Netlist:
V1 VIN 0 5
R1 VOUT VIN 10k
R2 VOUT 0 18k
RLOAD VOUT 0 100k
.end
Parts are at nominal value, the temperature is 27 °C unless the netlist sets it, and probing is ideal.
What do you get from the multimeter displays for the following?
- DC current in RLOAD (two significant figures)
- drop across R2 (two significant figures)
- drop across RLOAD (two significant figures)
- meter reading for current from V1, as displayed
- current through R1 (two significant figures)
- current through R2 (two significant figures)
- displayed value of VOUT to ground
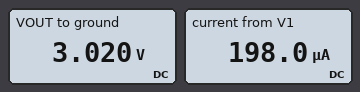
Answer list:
30 µA
3.0 V
3.0 V
198.0 µA
200 µA
170 µA
3.020 V
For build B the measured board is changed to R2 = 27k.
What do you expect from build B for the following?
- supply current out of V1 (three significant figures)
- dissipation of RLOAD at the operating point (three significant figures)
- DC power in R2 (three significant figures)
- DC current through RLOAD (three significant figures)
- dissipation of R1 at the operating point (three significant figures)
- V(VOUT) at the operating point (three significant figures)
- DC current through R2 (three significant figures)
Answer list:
160 µA
116 µW
428 µW
34.0 µA
256 µW
3.40 V
126 µA
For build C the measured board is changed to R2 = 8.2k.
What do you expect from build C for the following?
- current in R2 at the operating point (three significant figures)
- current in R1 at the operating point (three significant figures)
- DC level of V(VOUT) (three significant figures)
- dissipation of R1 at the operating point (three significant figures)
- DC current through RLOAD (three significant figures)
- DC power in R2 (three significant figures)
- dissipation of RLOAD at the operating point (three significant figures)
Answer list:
263 µA
284 µA
2.16 V
809 µW
21.6 µA
567 µW
46.5 µW
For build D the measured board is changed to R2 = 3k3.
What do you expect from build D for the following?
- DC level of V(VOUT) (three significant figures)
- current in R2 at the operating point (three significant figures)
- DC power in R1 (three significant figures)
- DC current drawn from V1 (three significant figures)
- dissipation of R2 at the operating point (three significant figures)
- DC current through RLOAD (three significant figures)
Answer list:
1.21 V
367 µA
1.44 mW
379 µA
444 µW
12.1 µA
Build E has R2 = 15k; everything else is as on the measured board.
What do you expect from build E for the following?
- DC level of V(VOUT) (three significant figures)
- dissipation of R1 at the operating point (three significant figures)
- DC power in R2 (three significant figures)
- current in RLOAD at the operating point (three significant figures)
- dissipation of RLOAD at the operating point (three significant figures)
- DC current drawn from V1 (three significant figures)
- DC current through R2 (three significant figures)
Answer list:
2.83 V
471 µW
534 µW
28.3 µA
80.1 µW
217 µA
189 µA
